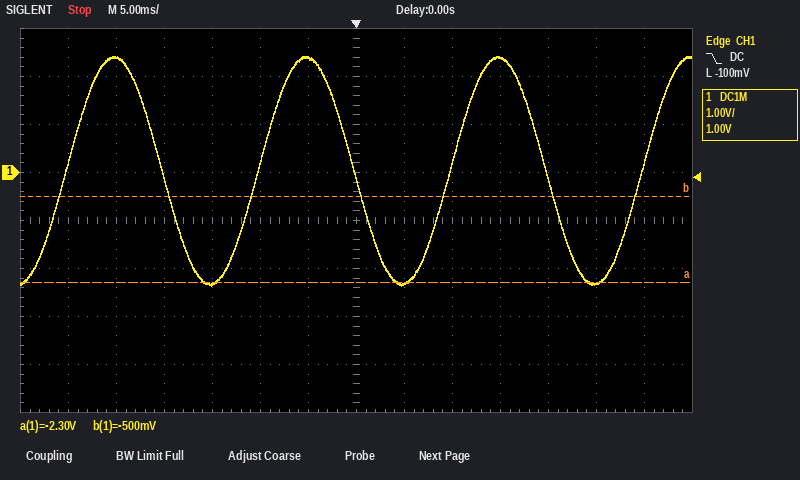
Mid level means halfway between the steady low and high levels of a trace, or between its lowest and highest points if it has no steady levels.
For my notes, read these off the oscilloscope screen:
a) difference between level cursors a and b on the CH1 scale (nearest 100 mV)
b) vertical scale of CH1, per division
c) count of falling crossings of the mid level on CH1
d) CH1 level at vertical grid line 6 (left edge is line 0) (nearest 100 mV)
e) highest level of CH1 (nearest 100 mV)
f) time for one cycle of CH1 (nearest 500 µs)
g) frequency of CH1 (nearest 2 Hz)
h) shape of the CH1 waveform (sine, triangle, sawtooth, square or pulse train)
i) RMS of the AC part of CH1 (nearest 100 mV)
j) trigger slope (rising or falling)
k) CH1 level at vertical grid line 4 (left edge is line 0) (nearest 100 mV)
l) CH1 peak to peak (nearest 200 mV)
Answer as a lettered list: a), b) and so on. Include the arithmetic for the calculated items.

a) 1.8 V
b) 1 V
c) 3
d) 2.4 V
e) 2.4 V
f) 20.0 ms
g) 1 / 20.0 ms ≈ 50 Hz
h) sine
i) 4.8 V / (2√2) ≈ 1.7 V
j) falling
k) -2.3 V
l) 4.8 V
